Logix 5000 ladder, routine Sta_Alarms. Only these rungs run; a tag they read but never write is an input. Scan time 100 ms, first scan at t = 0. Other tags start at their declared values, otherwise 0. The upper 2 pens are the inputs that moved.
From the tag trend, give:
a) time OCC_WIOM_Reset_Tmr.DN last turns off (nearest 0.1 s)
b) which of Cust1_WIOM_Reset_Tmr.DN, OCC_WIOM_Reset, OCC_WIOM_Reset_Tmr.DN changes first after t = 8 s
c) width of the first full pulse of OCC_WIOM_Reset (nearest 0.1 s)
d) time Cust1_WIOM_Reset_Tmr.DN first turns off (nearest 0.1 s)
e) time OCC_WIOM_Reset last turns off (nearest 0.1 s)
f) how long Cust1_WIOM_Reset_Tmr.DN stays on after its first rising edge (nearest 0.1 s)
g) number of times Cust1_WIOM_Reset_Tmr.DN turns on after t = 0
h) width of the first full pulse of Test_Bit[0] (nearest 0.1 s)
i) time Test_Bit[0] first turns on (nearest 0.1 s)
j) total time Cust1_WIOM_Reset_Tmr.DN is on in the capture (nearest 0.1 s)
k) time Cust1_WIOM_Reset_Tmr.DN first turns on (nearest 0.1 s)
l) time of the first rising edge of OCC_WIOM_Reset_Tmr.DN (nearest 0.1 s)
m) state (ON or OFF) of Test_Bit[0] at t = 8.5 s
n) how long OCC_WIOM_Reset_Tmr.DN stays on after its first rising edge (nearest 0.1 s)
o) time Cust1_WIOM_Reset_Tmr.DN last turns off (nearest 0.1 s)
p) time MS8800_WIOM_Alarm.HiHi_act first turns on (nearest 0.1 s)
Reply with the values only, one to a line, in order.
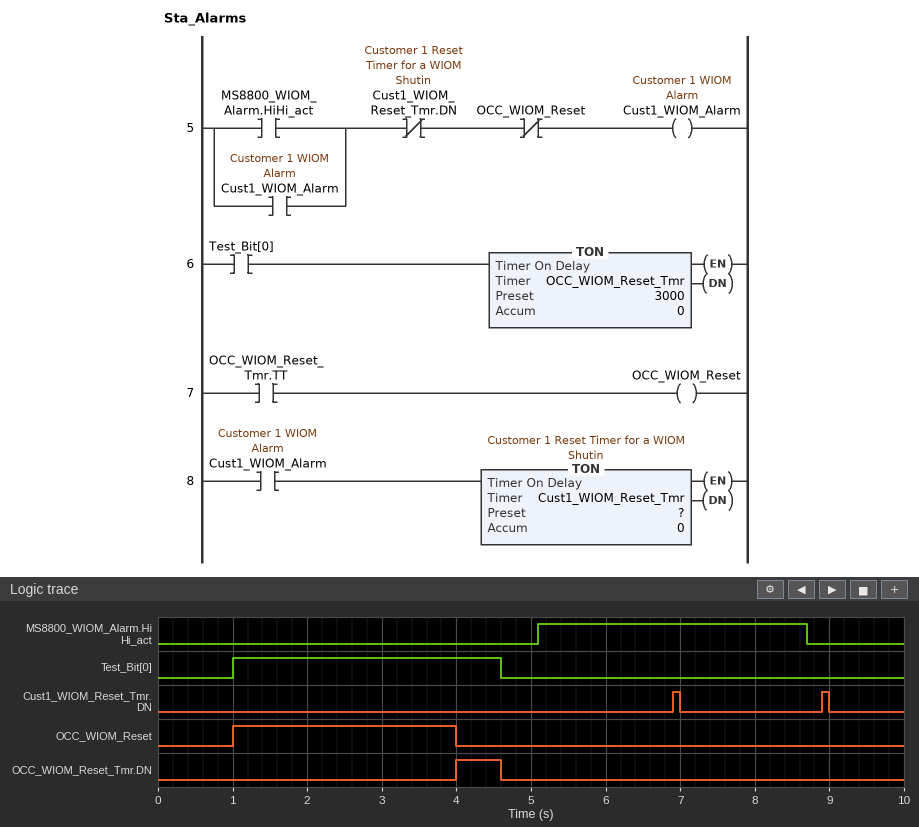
4.6 s
Cust1_WIOM_Reset_Tmr.DN
3.0 s
7.0 s
4.0 s
0.1 s
2
3.6 s
1.0 s
0.2 s
6.9 s
4.0 s
OFF
0.6 s
9.0 s
5.1 s
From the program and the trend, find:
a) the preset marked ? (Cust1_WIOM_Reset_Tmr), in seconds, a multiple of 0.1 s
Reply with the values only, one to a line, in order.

1.8 s
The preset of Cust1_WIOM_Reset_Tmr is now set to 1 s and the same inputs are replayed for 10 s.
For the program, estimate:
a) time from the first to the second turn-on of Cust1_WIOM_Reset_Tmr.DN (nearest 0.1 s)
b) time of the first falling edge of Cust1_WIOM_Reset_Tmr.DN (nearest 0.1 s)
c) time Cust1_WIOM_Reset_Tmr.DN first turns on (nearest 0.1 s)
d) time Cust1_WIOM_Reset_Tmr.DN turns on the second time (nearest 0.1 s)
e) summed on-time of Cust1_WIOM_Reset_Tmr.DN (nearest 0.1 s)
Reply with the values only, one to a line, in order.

1.2 s
6.2 s
6.1 s
7.3 s
0.3 s
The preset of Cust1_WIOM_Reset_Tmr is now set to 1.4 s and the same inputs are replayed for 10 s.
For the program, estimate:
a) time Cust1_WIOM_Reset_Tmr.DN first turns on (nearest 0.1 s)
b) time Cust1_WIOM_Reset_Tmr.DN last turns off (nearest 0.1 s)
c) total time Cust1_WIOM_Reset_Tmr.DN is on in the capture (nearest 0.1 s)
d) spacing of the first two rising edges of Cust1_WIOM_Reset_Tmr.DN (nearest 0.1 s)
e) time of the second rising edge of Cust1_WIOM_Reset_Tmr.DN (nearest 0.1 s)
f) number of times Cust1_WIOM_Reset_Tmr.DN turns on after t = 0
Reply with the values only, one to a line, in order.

6.5 s
9.8 s
0.3 s
1.6 s
8.1 s
3
